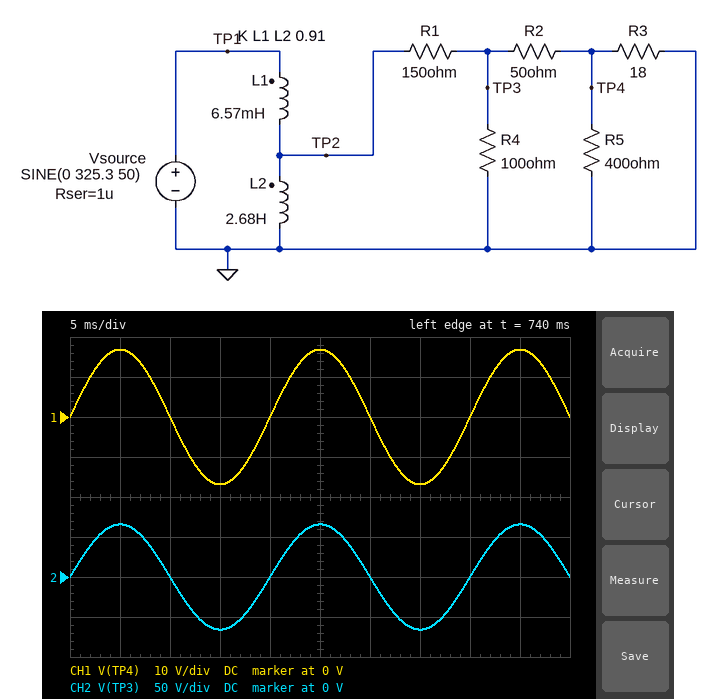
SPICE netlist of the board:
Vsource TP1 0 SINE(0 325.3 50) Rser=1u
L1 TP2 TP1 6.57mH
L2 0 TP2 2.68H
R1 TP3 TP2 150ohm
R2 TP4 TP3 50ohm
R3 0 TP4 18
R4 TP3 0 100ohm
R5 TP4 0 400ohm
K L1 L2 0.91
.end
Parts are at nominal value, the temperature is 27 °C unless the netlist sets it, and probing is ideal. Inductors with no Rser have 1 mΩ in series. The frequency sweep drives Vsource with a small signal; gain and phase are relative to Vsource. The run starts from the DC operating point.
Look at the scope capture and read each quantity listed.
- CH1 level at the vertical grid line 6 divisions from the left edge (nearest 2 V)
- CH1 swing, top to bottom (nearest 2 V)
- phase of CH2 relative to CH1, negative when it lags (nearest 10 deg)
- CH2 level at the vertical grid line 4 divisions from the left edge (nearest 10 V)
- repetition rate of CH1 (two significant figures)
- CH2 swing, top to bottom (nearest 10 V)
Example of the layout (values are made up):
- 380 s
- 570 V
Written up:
- 0 V
- 34 V
- 0 deg
- 0 V
- 50 Hz
- 130 V
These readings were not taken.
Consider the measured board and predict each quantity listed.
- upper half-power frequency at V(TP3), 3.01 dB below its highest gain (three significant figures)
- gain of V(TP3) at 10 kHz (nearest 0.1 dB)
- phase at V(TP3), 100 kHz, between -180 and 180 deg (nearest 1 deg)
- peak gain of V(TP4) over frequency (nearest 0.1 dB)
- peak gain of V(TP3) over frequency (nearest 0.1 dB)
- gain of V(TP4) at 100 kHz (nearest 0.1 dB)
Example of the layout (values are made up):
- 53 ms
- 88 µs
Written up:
- 29.3 kHz
- -14.4 dB
- -74 deg
- -25.7 dB
- -13.9 dB
- -36.7 dB
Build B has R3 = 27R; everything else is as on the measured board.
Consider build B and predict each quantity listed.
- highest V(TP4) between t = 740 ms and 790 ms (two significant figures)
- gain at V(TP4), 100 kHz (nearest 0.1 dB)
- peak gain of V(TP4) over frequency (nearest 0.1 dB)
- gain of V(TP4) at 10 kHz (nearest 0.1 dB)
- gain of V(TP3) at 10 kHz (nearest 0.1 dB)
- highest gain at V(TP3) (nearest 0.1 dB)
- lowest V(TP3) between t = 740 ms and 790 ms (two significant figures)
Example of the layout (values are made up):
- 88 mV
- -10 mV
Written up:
- 23 V
- -33.8 dB
- -22.9 dB
- -23.4 dB
- -13.9 dB
- -13.4 dB
- -69 V
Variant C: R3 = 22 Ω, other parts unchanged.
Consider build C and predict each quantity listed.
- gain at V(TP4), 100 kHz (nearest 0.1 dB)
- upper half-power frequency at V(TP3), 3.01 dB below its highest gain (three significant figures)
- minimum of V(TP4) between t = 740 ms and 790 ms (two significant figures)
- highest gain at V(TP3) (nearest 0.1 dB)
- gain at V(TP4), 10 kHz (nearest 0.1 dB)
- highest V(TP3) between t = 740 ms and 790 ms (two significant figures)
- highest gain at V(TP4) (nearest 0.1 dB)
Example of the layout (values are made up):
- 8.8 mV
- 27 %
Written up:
- -35.3 dB
- 29.5 kHz
- -20 V
- -13.7 dB
- -24.8 dB
- 67 V
- -24.3 dB
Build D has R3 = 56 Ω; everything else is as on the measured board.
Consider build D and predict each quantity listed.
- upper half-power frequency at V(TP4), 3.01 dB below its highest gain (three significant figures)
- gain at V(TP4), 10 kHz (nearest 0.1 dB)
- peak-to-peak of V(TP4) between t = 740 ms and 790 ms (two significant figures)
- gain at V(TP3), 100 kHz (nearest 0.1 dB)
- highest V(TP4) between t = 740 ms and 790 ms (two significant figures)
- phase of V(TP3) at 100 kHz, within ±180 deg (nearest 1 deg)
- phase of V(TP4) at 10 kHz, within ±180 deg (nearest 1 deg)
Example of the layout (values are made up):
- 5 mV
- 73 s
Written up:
- 30.8 kHz
- -19.0 dB
- 77 V
- -23.1 dB
- 38 V
- -73 deg
- -18 deg
